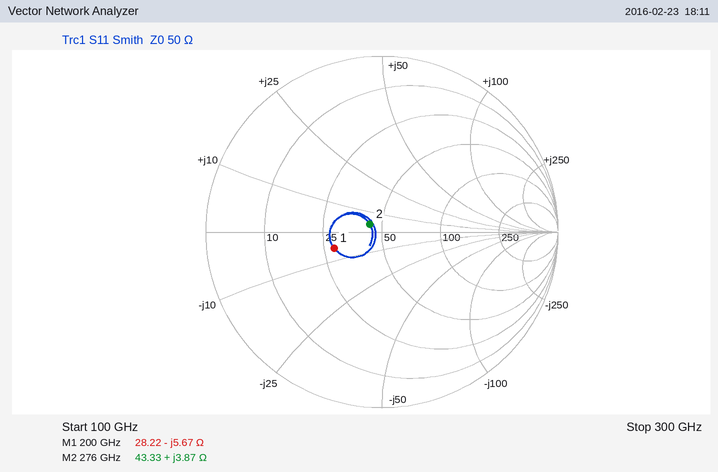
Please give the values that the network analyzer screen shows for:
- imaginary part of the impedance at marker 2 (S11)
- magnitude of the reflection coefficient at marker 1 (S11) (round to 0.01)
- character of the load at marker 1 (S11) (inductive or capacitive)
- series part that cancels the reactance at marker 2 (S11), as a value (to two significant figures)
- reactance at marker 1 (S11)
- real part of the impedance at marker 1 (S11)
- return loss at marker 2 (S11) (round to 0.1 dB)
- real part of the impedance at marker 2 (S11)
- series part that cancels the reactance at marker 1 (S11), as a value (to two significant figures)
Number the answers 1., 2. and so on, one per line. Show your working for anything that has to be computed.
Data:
1. +3.87 Ω
2. 0.29
3. capacitive
4. C = 1/(2π × 276 GHz × 3.87 Ω) ≈ 149 fF, so 150 fF to two significant figures
5. -5.67 Ω
6. 28.22 Ω
7. 21.7 dB
8. 43.33 Ω
9. L = 5.67 Ω/(2π × 200 GHz) ≈ 4.5 pH
